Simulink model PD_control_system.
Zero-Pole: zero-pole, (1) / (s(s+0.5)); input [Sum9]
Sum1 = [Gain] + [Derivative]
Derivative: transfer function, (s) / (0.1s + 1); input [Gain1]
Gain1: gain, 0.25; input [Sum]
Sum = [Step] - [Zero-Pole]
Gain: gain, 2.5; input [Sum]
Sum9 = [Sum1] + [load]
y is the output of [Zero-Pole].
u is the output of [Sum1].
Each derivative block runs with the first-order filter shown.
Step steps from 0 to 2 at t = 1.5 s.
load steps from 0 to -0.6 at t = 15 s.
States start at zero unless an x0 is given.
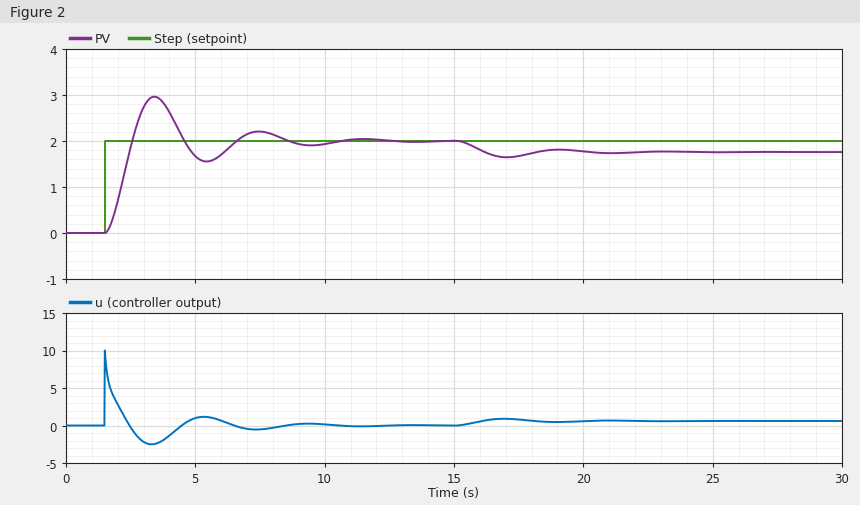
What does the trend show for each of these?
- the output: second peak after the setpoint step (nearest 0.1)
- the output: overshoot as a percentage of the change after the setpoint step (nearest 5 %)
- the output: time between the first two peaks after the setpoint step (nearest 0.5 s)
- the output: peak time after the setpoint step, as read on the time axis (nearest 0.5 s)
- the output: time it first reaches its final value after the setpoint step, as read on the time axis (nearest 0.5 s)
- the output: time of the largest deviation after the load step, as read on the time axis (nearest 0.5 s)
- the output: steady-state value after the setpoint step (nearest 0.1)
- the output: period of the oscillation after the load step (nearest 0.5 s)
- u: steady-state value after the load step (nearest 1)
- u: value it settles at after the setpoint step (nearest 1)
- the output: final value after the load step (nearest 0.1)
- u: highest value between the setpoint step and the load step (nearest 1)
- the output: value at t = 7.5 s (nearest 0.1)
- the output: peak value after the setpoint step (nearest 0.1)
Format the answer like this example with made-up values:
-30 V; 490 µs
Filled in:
2.2; 50 %; 4.0 s; 3.5 s; 2.5 s; 17.0 s; 2.0; 4.0 s; 1; 0; 1.8; 10; 2.2; 3.0
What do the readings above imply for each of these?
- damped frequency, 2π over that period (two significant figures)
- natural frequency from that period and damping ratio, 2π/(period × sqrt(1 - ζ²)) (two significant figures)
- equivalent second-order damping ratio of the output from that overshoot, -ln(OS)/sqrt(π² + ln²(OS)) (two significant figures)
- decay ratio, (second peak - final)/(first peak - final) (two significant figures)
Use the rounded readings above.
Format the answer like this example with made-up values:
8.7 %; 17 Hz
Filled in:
1.6 rad/s; 1.6 rad/s; 0.22; 0.20
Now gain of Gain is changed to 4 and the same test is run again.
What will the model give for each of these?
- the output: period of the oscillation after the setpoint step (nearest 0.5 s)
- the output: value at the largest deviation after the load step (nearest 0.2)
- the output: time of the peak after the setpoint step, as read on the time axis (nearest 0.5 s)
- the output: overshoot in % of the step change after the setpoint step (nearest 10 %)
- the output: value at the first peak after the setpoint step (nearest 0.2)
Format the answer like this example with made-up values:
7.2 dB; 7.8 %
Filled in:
3.0 s; 1.8; 3.0 s; 60 %; 3.2
